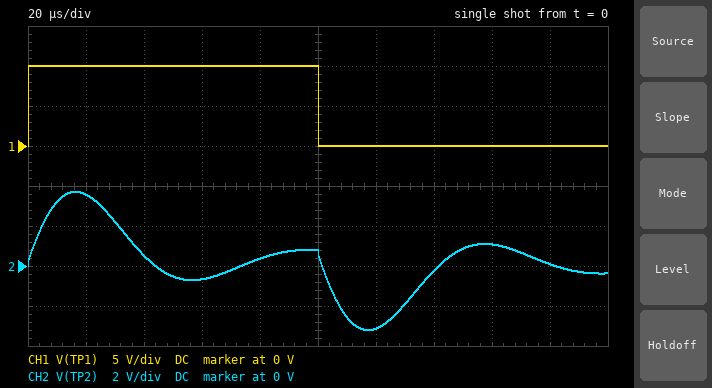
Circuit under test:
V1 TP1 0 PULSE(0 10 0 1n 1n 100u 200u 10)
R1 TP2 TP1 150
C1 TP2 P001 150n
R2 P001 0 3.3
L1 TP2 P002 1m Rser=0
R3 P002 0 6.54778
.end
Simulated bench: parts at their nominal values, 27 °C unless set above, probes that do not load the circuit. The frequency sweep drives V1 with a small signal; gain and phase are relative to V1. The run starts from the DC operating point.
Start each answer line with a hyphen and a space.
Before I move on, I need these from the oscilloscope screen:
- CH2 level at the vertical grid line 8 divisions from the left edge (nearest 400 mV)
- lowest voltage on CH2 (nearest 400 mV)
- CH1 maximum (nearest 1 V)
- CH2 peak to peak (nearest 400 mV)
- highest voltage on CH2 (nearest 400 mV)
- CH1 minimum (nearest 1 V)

- 1.2 V
- -3.2 V
- 10 V
- 6.8 V
- 3.6 V
- 0 V
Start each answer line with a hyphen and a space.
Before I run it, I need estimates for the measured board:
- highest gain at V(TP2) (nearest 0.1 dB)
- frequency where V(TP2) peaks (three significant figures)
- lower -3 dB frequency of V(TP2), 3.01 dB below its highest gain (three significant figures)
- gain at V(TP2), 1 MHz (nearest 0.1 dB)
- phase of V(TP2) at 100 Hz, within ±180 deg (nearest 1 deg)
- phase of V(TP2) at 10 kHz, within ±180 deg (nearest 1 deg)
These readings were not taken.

- -1.7 dB
- 13.1 kHz
- 9.55 kHz
- -32.9 dB
- 5 deg
- 36 deg
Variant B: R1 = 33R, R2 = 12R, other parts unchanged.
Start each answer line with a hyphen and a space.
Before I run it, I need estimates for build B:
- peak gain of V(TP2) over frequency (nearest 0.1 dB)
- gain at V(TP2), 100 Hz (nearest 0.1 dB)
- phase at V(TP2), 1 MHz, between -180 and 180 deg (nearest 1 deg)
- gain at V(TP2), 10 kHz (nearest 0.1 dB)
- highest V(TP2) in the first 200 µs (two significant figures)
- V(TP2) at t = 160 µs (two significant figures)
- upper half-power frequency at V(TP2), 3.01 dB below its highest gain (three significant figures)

- -0.7 dB
- -15.6 dB
- -4 deg
- -0.9 dB
- 7.3 V
- -820 mV
- 33.3 kHz
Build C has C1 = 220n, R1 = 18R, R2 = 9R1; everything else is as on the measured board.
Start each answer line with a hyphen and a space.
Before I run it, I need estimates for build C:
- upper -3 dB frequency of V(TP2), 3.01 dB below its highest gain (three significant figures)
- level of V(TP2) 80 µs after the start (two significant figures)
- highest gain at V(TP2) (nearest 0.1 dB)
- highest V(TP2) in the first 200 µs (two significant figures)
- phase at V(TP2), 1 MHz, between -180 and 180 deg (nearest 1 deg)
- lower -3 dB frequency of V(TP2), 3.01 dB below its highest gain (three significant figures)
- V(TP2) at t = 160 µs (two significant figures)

- 36.3 kHz
- 3.8 V
- -0.5 dB
- 8.2 V
- -3 deg
- 3.05 kHz
- -1.8 V
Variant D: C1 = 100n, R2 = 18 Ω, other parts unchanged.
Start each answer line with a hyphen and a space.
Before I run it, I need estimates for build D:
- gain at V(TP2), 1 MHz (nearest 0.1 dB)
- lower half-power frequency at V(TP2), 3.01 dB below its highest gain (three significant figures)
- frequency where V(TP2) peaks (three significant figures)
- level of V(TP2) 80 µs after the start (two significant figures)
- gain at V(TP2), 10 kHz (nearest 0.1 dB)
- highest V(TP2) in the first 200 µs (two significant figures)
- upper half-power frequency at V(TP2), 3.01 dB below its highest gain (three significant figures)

- -19.4 dB
- 10.2 kHz
- 15.4 kHz
- 590 mV
- -5.9 dB
- 3.9 V
- 23.6 kHz
